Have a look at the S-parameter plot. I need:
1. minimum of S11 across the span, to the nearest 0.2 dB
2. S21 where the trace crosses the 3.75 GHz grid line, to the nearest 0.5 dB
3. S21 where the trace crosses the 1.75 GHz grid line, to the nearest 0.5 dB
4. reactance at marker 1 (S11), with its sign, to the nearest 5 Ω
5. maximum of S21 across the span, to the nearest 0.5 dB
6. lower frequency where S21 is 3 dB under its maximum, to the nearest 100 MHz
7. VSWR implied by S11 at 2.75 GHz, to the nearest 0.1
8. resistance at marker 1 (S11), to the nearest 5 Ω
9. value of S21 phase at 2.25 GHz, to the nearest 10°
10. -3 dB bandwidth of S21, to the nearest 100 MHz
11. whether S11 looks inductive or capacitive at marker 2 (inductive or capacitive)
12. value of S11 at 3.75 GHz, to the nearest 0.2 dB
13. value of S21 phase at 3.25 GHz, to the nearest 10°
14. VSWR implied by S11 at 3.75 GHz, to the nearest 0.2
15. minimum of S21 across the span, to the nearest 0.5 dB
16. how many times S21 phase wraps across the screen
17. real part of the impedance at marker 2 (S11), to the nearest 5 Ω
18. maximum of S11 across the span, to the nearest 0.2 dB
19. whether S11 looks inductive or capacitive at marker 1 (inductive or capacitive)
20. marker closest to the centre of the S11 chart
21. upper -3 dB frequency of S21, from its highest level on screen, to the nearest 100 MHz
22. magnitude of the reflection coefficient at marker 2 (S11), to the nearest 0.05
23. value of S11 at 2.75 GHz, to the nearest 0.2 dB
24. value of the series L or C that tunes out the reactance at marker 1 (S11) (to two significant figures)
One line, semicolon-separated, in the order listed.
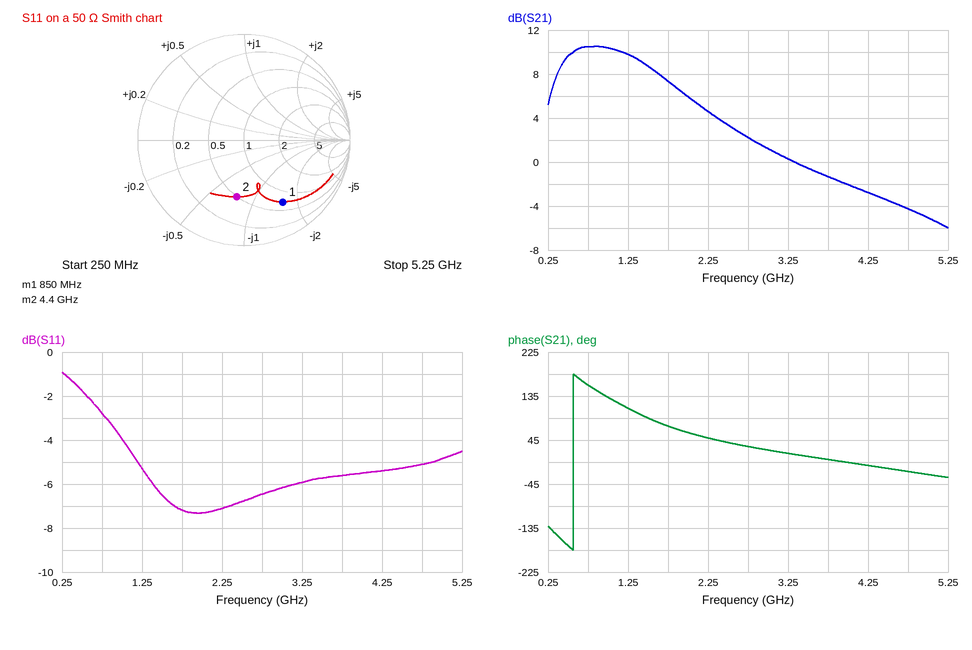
-7.4 dB; -1.5 dB; 7.5 dB; -80 Ω; 10.5 dB; 300 MHz; 2.8; 35 Ω; 50°; 1.4 GHz; capacitive; -5.6 dB; 20°; 3.2; -6.0 dB; 1; 25 Ω; -1.0 dB; capacitive; marker 2; 1.7 GHz; 0.55; -6.4 dB; 15 nH
